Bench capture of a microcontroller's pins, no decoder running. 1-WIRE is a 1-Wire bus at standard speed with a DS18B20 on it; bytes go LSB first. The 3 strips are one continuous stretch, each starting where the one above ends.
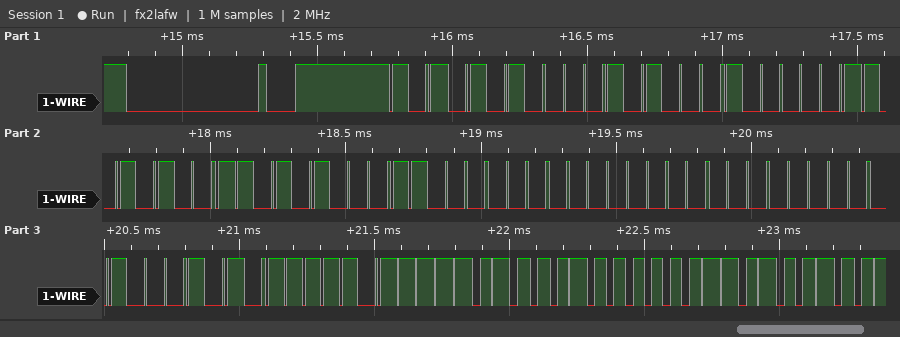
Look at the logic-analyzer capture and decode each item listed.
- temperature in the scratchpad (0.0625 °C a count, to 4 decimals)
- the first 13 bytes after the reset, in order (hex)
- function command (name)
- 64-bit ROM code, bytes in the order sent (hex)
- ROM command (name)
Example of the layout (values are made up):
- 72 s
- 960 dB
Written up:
- 34.9375 °C
- 55 28 82 95 15 03 00 00 A2 BE 2F 02 4B
- Read Scratchpad
- 28 82 95 15 03 00 00 A2
- Match ROM
